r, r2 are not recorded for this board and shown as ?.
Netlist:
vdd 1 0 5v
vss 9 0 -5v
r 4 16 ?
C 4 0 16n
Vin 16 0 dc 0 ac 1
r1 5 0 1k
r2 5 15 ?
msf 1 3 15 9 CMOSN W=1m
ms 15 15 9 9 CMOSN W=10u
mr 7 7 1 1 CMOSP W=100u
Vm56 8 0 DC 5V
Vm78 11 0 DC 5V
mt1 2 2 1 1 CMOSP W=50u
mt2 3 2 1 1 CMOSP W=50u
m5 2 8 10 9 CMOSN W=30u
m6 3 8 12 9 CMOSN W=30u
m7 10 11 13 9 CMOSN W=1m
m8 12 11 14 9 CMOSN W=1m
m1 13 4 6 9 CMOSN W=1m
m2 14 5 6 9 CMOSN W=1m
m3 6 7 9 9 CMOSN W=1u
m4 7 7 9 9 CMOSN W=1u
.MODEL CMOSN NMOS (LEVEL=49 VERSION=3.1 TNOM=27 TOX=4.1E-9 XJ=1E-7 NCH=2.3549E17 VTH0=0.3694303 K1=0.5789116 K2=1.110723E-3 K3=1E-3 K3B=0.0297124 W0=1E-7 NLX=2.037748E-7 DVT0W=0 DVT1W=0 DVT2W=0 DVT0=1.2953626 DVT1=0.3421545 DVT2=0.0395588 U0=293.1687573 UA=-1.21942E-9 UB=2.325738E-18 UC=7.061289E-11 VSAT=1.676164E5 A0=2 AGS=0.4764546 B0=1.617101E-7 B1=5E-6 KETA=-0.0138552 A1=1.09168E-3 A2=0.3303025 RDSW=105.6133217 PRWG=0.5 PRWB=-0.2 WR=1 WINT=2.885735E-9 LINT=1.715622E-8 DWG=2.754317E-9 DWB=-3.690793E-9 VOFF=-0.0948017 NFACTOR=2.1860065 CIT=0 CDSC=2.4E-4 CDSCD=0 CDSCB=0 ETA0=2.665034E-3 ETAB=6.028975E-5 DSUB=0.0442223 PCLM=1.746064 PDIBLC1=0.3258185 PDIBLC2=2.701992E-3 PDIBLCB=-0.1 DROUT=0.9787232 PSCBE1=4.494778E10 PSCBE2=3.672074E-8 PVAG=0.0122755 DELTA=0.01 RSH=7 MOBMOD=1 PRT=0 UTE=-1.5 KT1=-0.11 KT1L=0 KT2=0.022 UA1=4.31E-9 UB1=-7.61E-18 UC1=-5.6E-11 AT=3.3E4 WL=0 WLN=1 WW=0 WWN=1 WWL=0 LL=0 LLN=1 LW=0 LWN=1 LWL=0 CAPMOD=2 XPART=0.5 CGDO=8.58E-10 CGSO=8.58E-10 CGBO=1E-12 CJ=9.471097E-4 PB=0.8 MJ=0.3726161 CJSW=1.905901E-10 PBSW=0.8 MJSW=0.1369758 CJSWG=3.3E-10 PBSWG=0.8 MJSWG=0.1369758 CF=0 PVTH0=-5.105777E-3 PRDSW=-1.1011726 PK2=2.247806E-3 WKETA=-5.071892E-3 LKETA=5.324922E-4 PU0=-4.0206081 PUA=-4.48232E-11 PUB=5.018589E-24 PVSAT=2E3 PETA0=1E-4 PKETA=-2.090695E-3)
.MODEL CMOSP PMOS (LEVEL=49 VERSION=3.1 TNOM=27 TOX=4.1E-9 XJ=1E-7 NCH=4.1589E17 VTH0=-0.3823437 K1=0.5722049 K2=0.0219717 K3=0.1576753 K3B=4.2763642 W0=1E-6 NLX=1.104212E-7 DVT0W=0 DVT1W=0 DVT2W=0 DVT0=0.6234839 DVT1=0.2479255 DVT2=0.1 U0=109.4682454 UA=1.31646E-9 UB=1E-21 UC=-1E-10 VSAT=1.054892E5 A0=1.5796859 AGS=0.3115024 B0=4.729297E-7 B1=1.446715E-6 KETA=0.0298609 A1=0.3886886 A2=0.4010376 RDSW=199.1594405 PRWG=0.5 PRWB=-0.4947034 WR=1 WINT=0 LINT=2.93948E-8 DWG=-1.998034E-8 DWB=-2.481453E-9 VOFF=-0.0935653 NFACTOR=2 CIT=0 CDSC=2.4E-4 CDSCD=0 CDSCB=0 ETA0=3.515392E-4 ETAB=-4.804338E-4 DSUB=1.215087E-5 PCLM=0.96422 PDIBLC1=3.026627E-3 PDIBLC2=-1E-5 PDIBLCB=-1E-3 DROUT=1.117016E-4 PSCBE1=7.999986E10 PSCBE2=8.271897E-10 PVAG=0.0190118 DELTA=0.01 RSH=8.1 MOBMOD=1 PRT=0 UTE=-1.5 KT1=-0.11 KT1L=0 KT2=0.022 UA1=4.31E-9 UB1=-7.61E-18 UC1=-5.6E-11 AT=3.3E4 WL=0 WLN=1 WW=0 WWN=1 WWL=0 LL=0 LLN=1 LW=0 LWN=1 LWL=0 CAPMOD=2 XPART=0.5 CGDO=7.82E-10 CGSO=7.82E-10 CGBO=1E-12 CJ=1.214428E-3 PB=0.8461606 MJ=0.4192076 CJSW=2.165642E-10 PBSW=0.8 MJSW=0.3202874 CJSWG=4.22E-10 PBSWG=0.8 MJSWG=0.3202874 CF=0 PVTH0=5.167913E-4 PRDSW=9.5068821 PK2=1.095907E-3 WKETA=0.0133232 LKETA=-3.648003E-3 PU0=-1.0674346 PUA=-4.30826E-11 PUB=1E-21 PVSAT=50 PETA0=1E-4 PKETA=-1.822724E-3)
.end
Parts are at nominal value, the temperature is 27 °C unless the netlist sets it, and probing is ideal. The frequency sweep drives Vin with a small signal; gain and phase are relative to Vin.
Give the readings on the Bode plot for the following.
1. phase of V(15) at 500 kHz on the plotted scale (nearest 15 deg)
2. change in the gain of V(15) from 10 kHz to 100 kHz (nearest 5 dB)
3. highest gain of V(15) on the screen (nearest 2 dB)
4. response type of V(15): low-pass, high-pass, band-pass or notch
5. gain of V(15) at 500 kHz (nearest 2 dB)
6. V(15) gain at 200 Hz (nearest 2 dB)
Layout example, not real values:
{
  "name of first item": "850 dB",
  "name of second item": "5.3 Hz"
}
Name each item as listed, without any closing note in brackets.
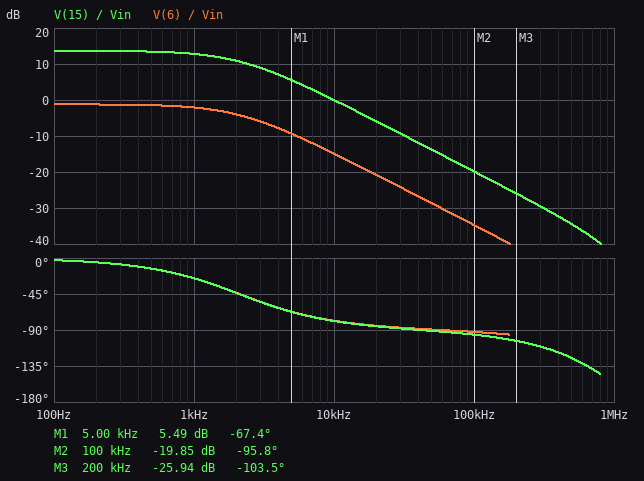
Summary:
{
  "phase of V(15) at 500 kHz on the plotted scale": "-120 deg",
  "change in the gain of V(15) from 10 kHz to 100 kHz": "-20 dB",
  "highest gain of V(15) on the screen": "14 dB",
  "response type of V(15): low-pass, high-pass, band-pass or notch": "low-pass",
  "gain of V(15) at 500 kHz": "-34 dB",
  "V(15) gain at 200 Hz": "14 dB"
}
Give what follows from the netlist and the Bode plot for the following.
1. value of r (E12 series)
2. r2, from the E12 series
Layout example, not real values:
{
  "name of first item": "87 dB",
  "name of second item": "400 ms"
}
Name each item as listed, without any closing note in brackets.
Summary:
{
  "value of r": "4.7 kΩ",
  "r2, from the E12 series": "3.9 kΩ"
}
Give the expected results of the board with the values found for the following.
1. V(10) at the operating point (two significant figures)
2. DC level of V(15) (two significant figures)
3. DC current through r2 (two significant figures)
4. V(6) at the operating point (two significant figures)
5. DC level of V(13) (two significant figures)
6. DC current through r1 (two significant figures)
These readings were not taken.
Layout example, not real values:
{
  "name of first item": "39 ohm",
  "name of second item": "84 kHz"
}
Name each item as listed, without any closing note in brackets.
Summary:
{
  "V(10) at the operating point": "3.1 V",
  "DC level of V(15)": "23 mV",
  "DC current through r2": "4.7 µA",
  "V(6) at the operating point": "-1.1 V",
  "DC level of V(13)": "3.1 V",
  "DC current through r1": "4.7 µA"
}
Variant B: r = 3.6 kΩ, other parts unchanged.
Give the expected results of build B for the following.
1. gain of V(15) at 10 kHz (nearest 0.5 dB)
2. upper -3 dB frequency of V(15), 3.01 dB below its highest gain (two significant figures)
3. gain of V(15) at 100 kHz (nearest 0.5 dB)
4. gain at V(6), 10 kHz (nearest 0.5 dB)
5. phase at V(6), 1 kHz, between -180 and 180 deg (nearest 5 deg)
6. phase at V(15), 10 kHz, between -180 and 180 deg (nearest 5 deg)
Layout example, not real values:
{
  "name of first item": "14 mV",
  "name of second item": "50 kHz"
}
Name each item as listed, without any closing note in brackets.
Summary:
{
  "gain of V(15) at 10 kHz": "2.0 dB",
  "upper -3 dB frequency of V(15), 3.01 dB below its highest gain": "2.8 kHz",
  "gain of V(15) at 100 kHz": "-17.5 dB",
  "gain at V(6), 10 kHz": "-12.5 dB",
  "phase at V(6), 1 kHz, between -180 and 180 deg": "-20 deg",
  "phase at V(15), 10 kHz, between -180 and 180 deg": "-75 deg"
}
